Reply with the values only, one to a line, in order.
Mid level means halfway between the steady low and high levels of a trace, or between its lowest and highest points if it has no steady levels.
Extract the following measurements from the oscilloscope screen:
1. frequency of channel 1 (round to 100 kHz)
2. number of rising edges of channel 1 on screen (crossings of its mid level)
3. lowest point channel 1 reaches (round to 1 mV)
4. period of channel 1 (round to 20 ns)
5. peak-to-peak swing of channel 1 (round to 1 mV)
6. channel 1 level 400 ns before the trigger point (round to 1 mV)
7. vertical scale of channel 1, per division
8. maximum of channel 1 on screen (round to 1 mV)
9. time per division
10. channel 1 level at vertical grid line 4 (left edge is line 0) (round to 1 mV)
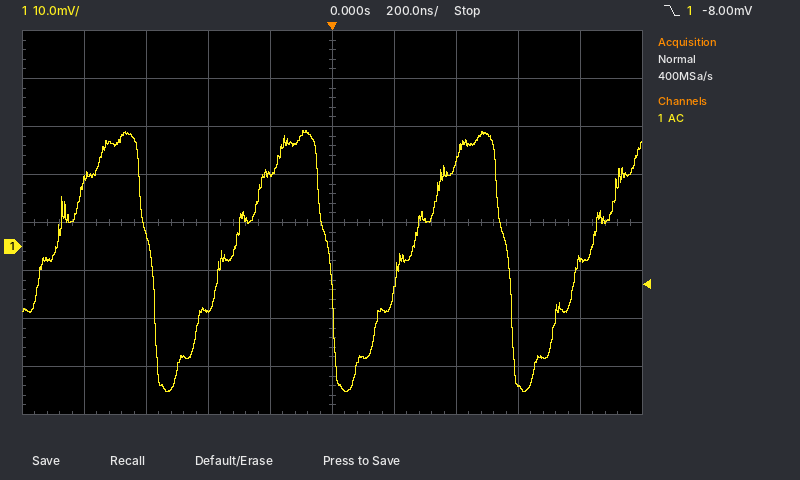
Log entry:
1.7 MHz
4
-30 mV
580 ns
54 mV
-13 mV
10 mV
24 mV
200 ns
15 mV
